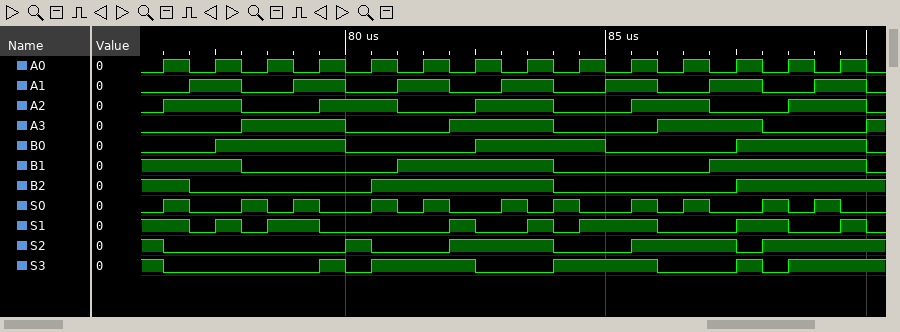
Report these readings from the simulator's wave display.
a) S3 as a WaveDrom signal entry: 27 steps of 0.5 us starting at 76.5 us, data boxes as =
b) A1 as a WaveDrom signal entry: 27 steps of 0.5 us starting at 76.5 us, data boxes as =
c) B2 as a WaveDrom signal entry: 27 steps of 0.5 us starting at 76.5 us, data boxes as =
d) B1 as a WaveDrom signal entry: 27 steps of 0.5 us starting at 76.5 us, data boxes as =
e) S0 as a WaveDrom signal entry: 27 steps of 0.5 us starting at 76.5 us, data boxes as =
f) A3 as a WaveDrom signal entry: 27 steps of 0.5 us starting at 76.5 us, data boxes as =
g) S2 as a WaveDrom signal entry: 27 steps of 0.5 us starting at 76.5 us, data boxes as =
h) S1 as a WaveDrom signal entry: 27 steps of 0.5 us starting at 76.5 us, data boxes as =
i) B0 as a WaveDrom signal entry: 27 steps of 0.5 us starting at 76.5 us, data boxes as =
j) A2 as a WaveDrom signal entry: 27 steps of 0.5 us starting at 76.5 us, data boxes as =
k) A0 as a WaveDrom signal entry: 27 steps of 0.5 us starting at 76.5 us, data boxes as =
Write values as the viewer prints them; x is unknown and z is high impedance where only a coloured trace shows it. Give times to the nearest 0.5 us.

{name: 'S3', wave: '0.....101...0..1...0..101..'}
{name: 'A1', wave: '01.0.1.0.1.0.1.0.1.0.1.0.1.'}
{name: 'B2', wave: '10......1......0......1....'}
{name: 'B1', wave: '1..0.....1.....0.....1.....'}
{name: 'S0', wave: '10.1010.1010.1010.1010.1010'}
{name: 'A3', wave: '0..1...0...1...0...1...0...'}
{name: 'S2', wave: '0......10..1...0..1...01...'}
{name: 'S1', wave: '10101.0....10.101..0..1.0.1'}
{name: 'B0', wave: '0.1....0....1....0....1....'}
{name: 'A2', wave: '1..0..1..0..1..0..1..0..1..'}
{name: 'A0', wave: '101010101010101010101010101'}
